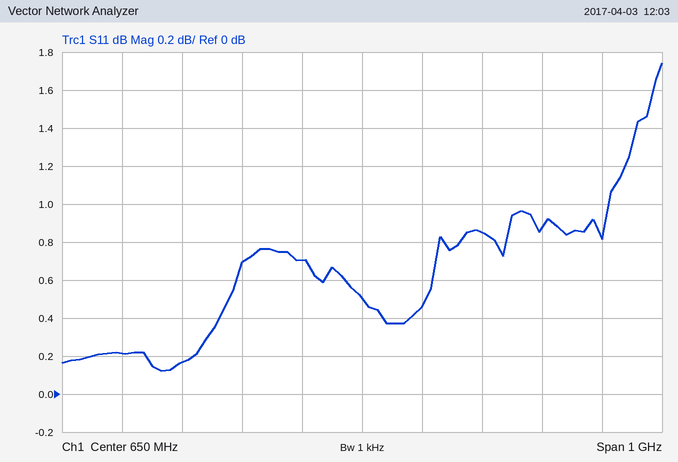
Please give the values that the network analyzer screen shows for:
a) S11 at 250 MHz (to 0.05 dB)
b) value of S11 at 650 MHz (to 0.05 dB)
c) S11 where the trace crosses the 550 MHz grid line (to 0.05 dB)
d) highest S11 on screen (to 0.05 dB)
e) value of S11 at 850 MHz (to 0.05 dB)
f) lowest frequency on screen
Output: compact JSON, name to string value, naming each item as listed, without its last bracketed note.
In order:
{"S11 at 250 MHz": "0.20 dB", "value of S11 at 650 MHz": "0.50 dB", "S11 where the trace crosses the 550 MHz grid line": "0.70 dB", "highest S11 on screen": "1.75 dB", "value of S11 at 850 MHz": "0.85 dB", "lowest frequency on screen": "150 MHz"}
